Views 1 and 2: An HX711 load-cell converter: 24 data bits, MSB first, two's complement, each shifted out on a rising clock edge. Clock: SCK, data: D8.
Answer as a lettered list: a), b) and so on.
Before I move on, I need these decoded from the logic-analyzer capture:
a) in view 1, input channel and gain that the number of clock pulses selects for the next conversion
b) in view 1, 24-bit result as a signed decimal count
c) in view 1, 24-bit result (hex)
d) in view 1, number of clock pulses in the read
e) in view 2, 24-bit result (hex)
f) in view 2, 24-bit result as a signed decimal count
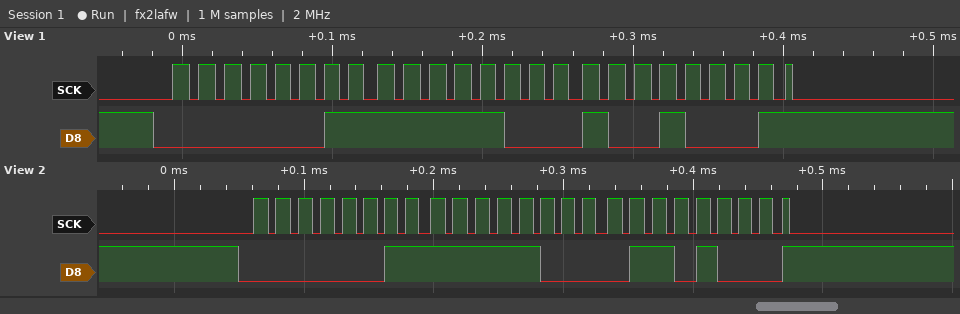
a) channel A, gain 128
b) 260241
c) 0x03F891
d) 25
e) 0x03F868
f) 260200
